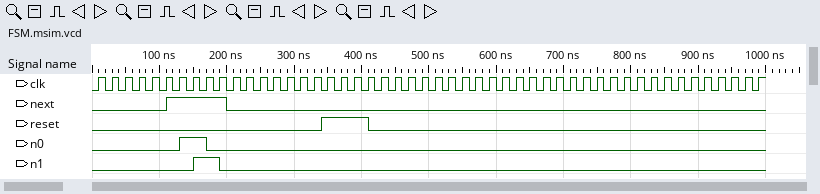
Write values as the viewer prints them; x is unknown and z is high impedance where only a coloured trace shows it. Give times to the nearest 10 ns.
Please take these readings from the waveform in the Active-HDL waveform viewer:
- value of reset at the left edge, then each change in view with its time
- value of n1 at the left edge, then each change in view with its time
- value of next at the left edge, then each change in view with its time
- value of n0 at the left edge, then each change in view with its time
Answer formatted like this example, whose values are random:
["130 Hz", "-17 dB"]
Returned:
["0, 1 at 340 ns, 0 at 410 ns", "0, 1 at 150 ns, 0 at 190 ns", "0, 1 at 110 ns, 0 at 200 ns", "0, 1 at 130 ns, 0 at 170 ns"]
